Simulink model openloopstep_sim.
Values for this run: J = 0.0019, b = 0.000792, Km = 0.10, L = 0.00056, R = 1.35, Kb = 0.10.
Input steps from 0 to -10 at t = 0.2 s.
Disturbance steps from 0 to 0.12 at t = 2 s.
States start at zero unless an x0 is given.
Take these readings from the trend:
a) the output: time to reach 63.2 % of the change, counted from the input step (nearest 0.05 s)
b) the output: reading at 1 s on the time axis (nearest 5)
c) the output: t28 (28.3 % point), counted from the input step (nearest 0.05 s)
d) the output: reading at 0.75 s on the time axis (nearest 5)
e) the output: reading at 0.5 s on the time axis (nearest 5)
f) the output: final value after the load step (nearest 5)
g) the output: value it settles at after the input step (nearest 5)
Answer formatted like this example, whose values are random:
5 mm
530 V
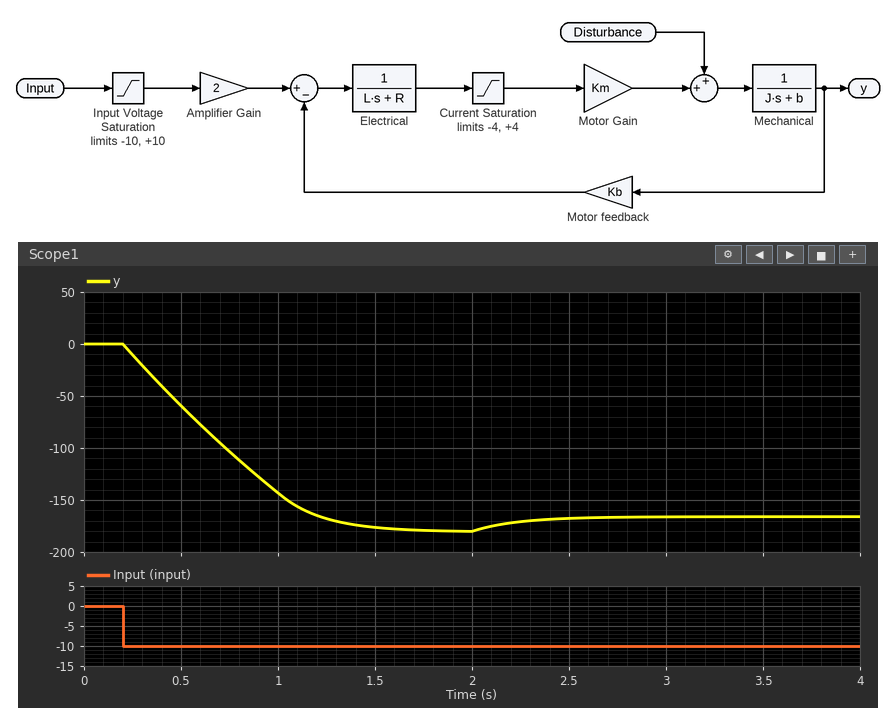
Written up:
0.60 s
-145
0.25 s
-105
-60
-165
-180
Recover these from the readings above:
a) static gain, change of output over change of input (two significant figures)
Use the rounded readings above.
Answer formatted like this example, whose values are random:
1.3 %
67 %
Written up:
18
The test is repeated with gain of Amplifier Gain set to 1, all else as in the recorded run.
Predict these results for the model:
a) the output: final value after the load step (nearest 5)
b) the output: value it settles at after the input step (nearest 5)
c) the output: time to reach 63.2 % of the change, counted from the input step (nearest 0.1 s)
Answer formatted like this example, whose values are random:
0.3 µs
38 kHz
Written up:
-75
-90
0.3 s
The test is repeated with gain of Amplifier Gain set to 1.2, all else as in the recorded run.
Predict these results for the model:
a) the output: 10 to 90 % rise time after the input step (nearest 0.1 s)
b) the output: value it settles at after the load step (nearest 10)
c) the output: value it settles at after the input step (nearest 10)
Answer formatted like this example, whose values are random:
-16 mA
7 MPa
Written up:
0.6 s
-90
-110
